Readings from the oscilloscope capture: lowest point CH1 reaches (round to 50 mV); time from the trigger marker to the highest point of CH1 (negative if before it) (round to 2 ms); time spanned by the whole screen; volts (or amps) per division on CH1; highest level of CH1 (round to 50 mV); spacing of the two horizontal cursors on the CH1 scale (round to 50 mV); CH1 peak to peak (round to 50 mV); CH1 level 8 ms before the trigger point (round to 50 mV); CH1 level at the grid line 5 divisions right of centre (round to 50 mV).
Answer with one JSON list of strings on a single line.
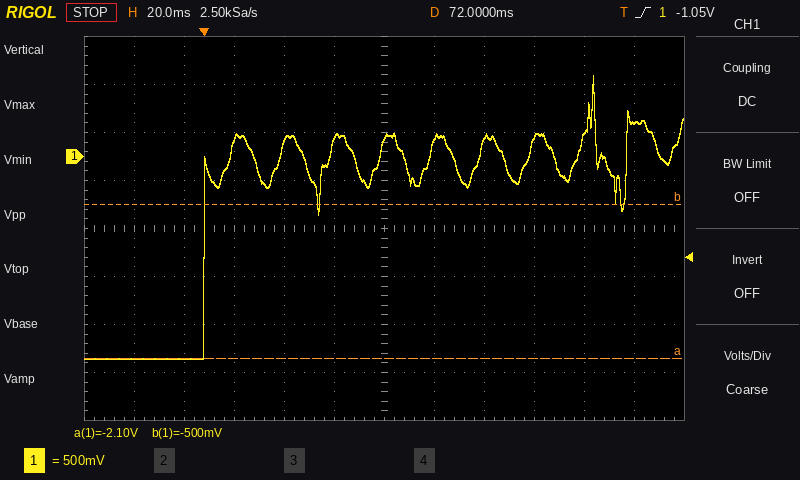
["-2.10 V", "+156 ms", "240 ms", "500 mV", "850 mV", "1.60 V", "2.95 V", "-2.10 V", "350 mV"]
